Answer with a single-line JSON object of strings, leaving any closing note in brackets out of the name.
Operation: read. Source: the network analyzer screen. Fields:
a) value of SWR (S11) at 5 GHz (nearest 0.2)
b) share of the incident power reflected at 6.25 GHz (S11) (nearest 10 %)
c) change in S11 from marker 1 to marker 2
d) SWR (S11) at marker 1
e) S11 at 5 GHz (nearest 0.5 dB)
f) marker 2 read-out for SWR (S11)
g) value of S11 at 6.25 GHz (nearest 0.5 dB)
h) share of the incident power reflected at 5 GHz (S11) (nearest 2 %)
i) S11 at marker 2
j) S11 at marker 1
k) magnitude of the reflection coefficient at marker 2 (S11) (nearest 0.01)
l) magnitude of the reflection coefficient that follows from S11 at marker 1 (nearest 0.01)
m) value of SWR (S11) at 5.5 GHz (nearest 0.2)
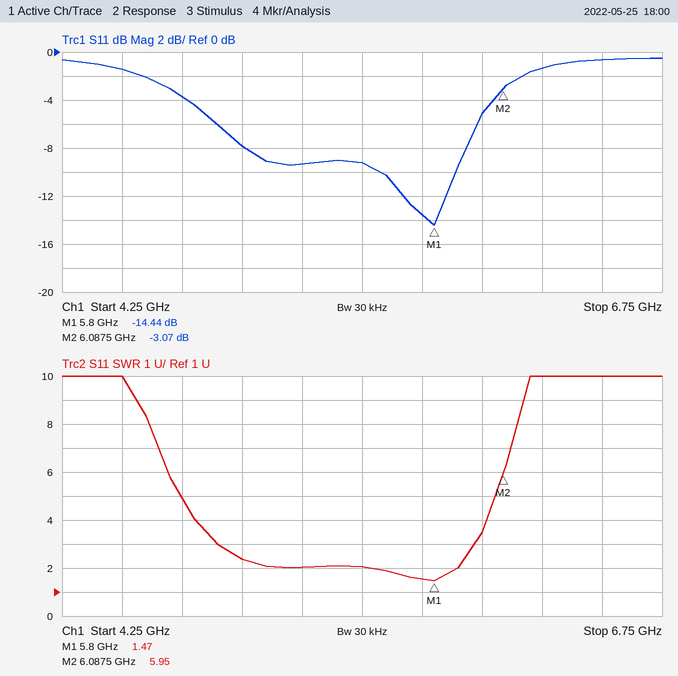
{"value of SWR (S11) at 5 GHz": "2.4", "share of the incident power reflected at 6.25 GHz (S11)": "70 %", "change in S11 from marker 1 to marker 2": "11.37 dB", "SWR (S11) at marker 1": "1.47", "S11 at 5 GHz": "-8.0 dB", "marker 2 read-out for SWR": "5.95", "value of S11 at 6.25 GHz": "-1.5 dB", "share of the incident power reflected at 5 GHz (S11)": "16 %", "S11 at marker 2": "-3.07 dB", "S11 at marker 1": "-14.44 dB", "magnitude of the reflection coefficient at marker 2 (S11)": "0.70", "magnitude of the reflection coefficient that follows from S11 at marker 1": "0.19", "value of SWR (S11) at 5.5 GHz": "2.0"}
